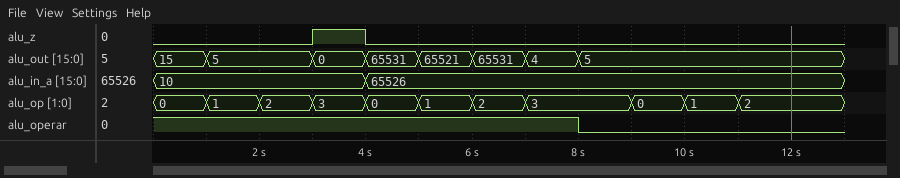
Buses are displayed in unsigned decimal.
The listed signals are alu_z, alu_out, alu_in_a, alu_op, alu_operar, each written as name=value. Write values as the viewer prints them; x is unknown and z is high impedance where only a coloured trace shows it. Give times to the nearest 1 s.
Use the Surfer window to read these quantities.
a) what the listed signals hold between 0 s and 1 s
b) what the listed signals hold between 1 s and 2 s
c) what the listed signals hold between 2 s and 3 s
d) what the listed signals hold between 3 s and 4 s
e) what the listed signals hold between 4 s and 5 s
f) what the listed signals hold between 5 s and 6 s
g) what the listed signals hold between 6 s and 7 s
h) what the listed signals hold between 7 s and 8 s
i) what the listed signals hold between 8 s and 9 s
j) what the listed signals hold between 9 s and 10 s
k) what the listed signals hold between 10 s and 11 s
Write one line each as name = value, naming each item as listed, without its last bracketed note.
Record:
what the listed signals hold between 0 s and 1 s = alu_z=0, alu_out=15, alu_in_a=10, alu_op=0, alu_operar=1
what the listed signals hold between 1 s and 2 s = alu_z=0, alu_out=5, alu_in_a=10, alu_op=1, alu_operar=1
what the listed signals hold between 2 s and 3 s = alu_z=0, alu_out=5, alu_in_a=10, alu_op=2, alu_operar=1
what the listed signals hold between 3 s and 4 s = alu_z=1, alu_out=0, alu_in_a=10, alu_op=3, alu_operar=1
what the listed signals hold between 4 s and 5 s = alu_z=0, alu_out=65531, alu_in_a=65526, alu_op=0, alu_operar=1
what the listed signals hold between 5 s and 6 s = alu_z=0, alu_out=65521, alu_in_a=65526, alu_op=1, alu_operar=1
what the listed signals hold between 6 s and 7 s = alu_z=0, alu_out=65531, alu_in_a=65526, alu_op=2, alu_operar=1
what the listed signals hold between 7 s and 8 s = alu_z=0, alu_out=4, alu_in_a=65526, alu_op=3, alu_operar=1
what the listed signals hold between 8 s and 9 s = alu_z=0, alu_out=5, alu_in_a=65526, alu_op=3, alu_operar=0
what the listed signals hold between 9 s and 10 s = alu_z=0, alu_out=5, alu_in_a=65526, alu_op=0, alu_operar=0
what the listed signals hold between 10 s and 11 s = alu_z=0, alu_out=5, alu_in_a=65526, alu_op=1, alu_operar=0
